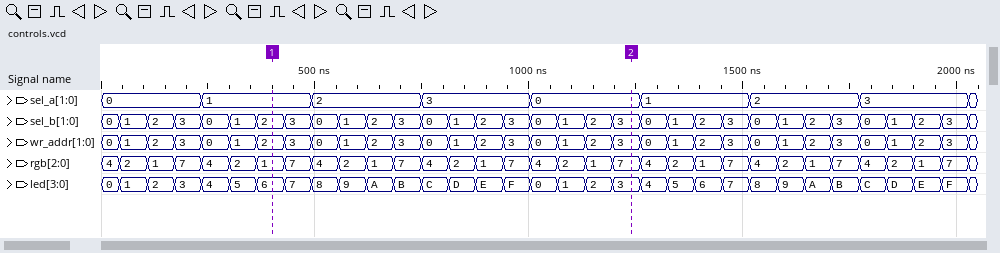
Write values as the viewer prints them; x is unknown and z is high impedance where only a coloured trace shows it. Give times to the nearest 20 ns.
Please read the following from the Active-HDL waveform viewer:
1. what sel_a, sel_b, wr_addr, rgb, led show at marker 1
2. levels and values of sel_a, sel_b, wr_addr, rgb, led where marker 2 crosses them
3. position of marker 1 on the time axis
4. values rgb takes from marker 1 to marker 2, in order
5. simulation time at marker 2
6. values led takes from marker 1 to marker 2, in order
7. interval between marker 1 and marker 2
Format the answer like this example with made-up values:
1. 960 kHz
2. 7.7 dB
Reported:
1. sel_a=1, sel_b=2, wr_addr=2, rgb=1, led=6
2. sel_a=0, sel_b=3, wr_addr=3, rgb=7, led=3
3. 400 ns
4. 1, 7, 4, 2, 1, 7, 4, 2, 1, 7, 4, 2, 1, 7
5. 1240 ns
6. 6, 7, 8, 9, A, B, C, D, E, F, 0, 1, 2, 3
7. 840 ns
